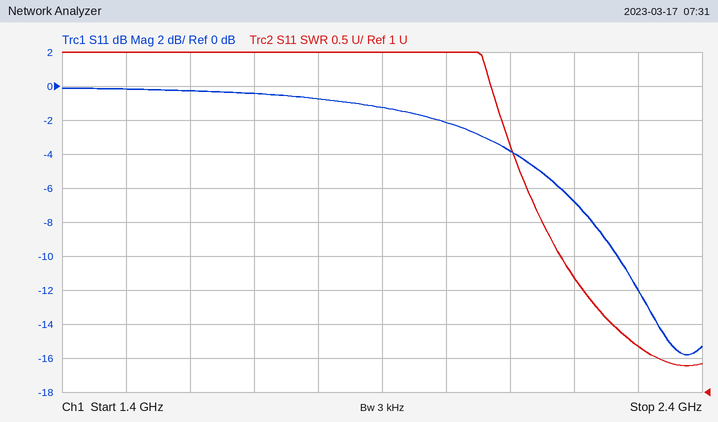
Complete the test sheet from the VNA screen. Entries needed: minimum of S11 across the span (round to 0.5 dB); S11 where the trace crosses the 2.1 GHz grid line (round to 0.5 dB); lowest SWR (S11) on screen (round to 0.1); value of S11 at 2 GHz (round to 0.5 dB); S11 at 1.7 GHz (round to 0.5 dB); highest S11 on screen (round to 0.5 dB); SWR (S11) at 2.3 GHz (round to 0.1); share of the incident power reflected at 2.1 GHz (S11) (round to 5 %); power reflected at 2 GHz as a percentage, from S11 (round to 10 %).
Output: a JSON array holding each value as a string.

["-16.0 dB", "-4.0 dB", "1.4", "-2.0 dB", "-0.5 dB", "0.0 dB", "1.7", "40 %", "60 %"]
